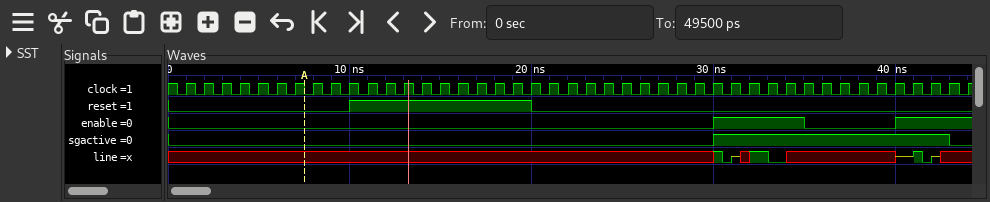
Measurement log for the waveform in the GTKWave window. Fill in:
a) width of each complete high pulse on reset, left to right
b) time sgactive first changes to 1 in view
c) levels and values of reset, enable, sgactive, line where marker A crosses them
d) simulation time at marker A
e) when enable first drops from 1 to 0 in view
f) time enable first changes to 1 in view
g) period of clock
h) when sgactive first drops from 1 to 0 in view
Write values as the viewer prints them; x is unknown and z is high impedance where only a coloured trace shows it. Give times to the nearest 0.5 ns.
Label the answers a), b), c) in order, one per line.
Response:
a) 10 ns
b) 30 ns
c) reset=0, enable=0, sgactive=0, line=x
d) 7.5 ns
e) 35 ns
f) 30 ns
g) 1 ns
h) 43 ns
